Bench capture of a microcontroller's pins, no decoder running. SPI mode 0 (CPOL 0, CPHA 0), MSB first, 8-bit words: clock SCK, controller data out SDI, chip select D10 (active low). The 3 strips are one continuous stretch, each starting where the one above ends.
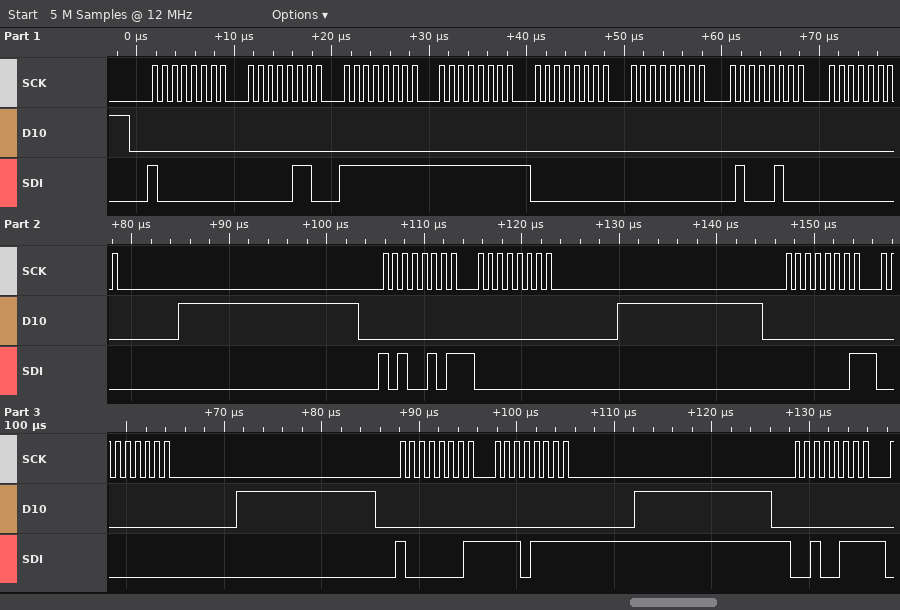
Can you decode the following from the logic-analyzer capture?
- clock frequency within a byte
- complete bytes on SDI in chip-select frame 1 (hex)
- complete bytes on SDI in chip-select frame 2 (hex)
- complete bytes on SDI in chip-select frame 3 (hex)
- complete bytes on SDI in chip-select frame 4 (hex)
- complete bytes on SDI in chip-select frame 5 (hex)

1 MHz
80 06 FF FF 00 00 44 00
A5 00
01 00
81 EF
27
